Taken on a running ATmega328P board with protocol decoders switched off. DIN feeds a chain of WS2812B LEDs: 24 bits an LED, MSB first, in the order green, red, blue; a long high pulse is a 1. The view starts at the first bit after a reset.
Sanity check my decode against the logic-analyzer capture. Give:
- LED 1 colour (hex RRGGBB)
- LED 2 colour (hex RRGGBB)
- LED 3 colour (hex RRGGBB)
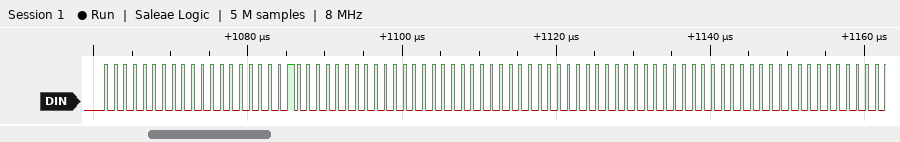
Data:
#000010
#000000
#000000
